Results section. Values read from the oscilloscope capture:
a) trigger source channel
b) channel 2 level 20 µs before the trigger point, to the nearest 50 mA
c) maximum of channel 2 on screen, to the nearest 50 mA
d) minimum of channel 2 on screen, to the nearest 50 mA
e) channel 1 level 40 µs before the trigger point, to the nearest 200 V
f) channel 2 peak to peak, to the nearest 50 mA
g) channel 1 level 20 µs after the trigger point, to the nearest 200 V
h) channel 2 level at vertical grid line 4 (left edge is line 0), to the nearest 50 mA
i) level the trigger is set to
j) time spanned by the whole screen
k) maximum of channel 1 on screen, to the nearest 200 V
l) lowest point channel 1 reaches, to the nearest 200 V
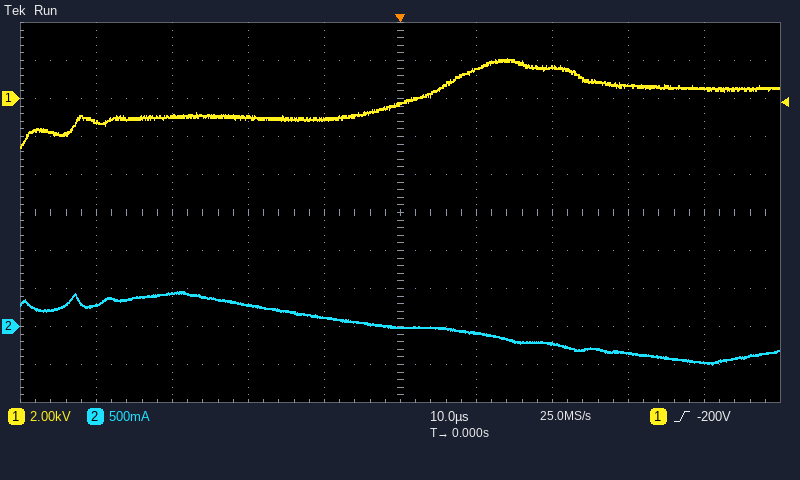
channel 1
300 mA
450 mA
-500 mA
-1.2 kV
950 mA
1.6 kV
100 mA
-200 V
100 µs
2.2 kV
-2.6 kV
